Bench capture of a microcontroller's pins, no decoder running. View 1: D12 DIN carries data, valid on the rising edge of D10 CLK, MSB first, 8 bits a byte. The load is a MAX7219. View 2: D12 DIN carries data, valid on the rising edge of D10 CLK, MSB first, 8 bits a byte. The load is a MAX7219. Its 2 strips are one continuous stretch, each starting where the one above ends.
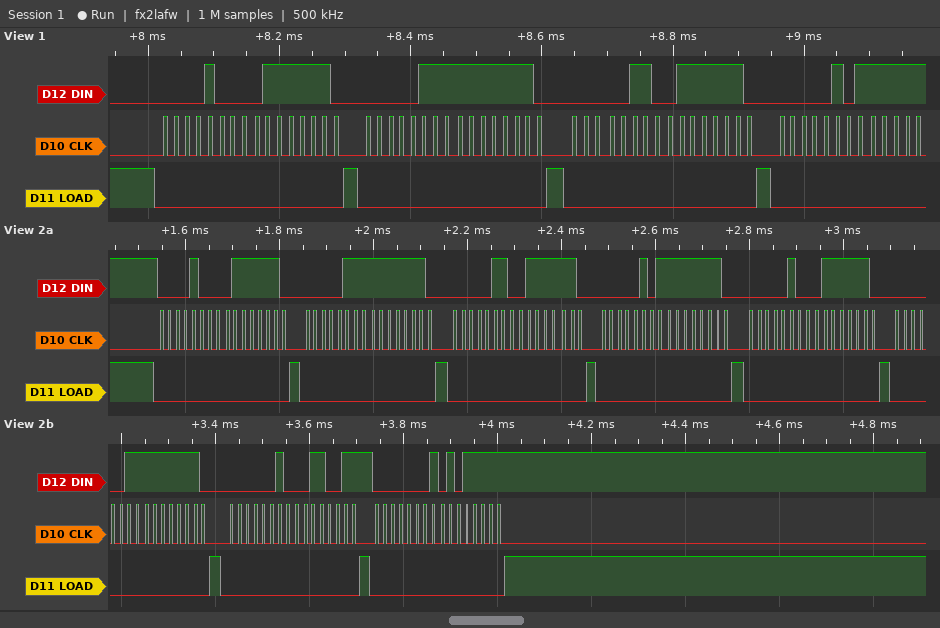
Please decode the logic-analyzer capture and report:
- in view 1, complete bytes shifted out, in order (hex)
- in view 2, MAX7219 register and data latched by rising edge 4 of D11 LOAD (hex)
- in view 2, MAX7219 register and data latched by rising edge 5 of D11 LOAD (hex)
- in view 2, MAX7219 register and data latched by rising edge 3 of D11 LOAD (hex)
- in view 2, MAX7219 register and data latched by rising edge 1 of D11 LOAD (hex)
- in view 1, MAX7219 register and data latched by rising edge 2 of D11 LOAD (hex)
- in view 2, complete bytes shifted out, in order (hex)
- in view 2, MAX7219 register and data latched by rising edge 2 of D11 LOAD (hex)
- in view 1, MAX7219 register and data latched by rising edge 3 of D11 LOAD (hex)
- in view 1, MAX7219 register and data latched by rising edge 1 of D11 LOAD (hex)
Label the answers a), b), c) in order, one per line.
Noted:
a) 08 7E 07 FE 06 7E 05
b) register 0x5, data 0xFE
c) register 0x4, data 0x7E
d) register 0x6, data 0x7E
e) register 0x8, data 0x7E
f) register 0x7, data 0xFE
g) 08 7E 07 FE 06 7E 05 FE 04 7E 03 FE 02 33 01 5F
h) register 0x7, data 0xFE
i) register 0x6, data 0x7E
j) register 0x8, data 0x7E
